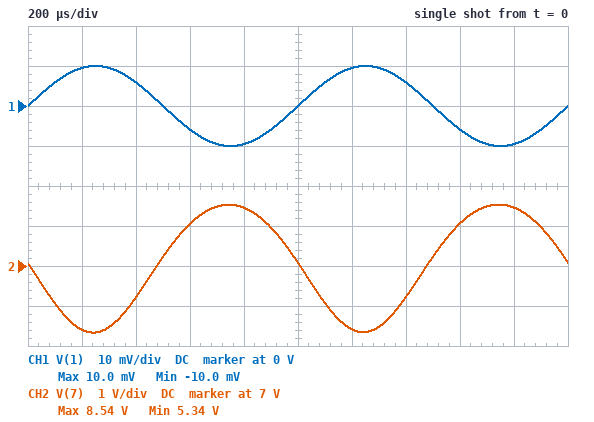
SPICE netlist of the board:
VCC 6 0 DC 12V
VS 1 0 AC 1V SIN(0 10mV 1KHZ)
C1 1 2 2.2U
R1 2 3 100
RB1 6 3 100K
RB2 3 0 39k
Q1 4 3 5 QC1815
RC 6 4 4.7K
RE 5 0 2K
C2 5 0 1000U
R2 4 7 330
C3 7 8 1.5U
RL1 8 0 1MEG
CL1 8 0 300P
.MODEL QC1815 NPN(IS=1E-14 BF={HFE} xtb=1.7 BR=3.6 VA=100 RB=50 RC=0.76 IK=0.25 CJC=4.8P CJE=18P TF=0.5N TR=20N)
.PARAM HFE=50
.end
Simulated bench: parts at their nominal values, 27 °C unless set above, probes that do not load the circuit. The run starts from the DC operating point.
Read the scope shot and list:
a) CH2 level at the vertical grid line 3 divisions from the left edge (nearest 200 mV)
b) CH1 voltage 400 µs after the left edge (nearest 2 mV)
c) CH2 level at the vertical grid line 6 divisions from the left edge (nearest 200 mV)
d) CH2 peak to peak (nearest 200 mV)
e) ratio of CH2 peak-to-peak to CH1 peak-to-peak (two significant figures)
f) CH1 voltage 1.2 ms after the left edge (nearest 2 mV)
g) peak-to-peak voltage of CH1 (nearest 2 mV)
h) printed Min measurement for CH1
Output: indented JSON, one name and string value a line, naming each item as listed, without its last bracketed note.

{
  "CH2 level at the vertical grid line 3 divisions from the left edge": "8.0 V",
  "CH1 voltage 400 µs after the left edge": "6 mV",
  "CH2 level at the vertical grid line 6 divisions from the left edge": "5.4 V",
  "CH2 peak to peak": "3.2 V",
  "ratio of CH2 peak-to-peak to CH1 peak-to-peak": "160",
  "CH1 voltage 1.2 ms after the left edge": "10 mV",
  "peak-to-peak voltage of CH1": "20 mV",
  "printed Min measurement for CH1": "-10.0 mV"
}
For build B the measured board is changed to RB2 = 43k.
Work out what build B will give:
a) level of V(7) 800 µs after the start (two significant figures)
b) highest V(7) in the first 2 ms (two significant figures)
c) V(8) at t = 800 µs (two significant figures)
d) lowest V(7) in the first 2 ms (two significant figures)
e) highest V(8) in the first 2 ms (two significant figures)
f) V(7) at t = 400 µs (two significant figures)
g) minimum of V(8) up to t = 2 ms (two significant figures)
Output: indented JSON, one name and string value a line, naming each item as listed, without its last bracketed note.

{
  "level of V(7) 800 µs after the start": "8.2 V",
  "highest V(7) in the first 2 ms": "8.3 V",
  "V(8) at t = 800 µs": "1.5 V",
  "lowest V(7) in the first 2 ms": "4.9 V",
  "highest V(8) in the first 2 ms": "1.6 V",
  "V(7) at t = 400 µs": "5.8 V",
  "minimum of V(8) up to t = 2 ms": "-1.8 V"
}
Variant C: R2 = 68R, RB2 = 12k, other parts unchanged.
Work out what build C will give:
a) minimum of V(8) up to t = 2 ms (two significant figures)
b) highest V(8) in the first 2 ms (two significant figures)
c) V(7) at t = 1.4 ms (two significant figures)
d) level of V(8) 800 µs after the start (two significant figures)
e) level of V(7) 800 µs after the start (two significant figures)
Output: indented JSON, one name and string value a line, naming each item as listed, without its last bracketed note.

{
  "minimum of V(8) up to t = 2 ms": "-590 mV",
  "highest V(8) in the first 2 ms": "440 mV",
  "V(7) at t = 1.4 ms": "10 V",
  "level of V(8) 800 µs after the start": "420 mV",
  "level of V(7) 800 µs after the start": "11 V"
}
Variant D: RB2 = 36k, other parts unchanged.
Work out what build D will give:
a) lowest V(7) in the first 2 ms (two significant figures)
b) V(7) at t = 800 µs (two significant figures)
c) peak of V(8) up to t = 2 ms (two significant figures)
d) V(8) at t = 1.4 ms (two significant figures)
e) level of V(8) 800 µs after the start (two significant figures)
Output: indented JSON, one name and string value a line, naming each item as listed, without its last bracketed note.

{
  "lowest V(7) in the first 2 ms": "5.7 V",
  "V(7) at t = 800 µs": "8.7 V",
  "peak of V(8) up to t = 2 ms": "1.4 V",
  "V(8) at t = 1.4 ms": "-800 mV",
  "level of V(8) 800 µs after the start": "1.3 V"
}
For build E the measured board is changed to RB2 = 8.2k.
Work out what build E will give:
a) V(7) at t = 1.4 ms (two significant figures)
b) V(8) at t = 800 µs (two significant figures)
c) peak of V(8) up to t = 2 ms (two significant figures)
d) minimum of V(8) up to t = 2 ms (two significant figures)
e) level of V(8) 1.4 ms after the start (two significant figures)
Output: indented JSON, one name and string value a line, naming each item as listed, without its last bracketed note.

{
  "V(7) at t = 1.4 ms": "11 V",
  "V(8) at t = 800 µs": "200 mV",
  "peak of V(8) up to t = 2 ms": "210 mV",
  "minimum of V(8) up to t = 2 ms": "-290 mV",
  "level of V(8) 1.4 ms after the start": "-150 mV"
}
